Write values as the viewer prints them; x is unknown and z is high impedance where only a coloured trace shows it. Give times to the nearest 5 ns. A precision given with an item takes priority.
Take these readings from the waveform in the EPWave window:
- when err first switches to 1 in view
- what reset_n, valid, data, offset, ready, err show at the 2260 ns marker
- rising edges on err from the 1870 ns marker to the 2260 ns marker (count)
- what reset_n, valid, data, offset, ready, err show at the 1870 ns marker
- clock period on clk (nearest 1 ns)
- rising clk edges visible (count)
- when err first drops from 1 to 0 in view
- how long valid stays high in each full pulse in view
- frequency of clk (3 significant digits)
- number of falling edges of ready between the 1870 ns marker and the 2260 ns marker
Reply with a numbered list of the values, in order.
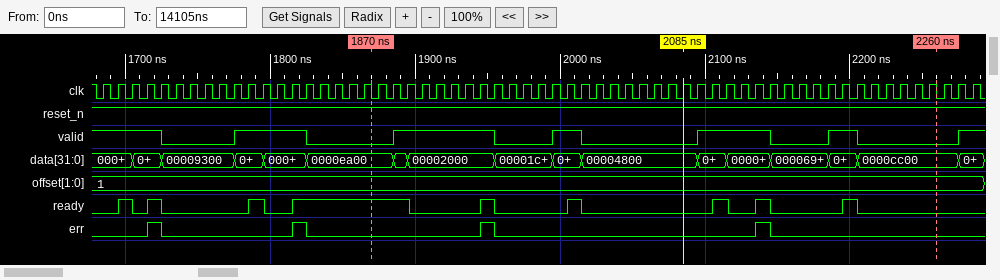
1. 1715 ns
2. reset_n=1, valid=0, data=0000cc00, offset=1, ready=0, err=0
3. 2
4. reset_n=1, valid=0, data=0000ea00, offset=1, ready=1, err=0
5. 10 ns
6. 61
7. 1725 ns
8. 50 ns, 70 ns, 20 ns, 50 ns, 20 ns
9. 100 MHz
10. 6
